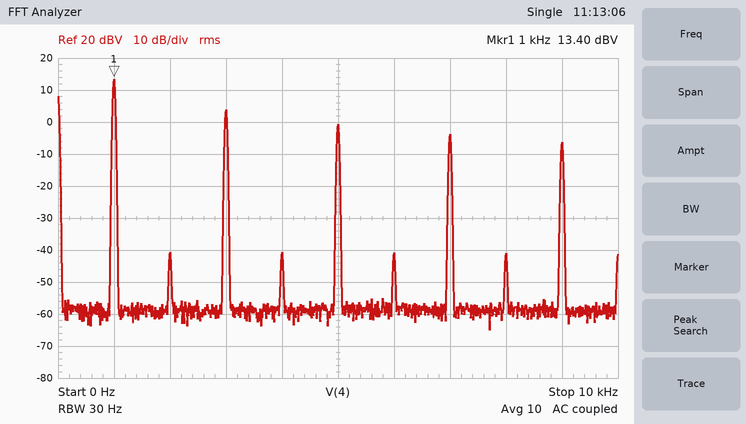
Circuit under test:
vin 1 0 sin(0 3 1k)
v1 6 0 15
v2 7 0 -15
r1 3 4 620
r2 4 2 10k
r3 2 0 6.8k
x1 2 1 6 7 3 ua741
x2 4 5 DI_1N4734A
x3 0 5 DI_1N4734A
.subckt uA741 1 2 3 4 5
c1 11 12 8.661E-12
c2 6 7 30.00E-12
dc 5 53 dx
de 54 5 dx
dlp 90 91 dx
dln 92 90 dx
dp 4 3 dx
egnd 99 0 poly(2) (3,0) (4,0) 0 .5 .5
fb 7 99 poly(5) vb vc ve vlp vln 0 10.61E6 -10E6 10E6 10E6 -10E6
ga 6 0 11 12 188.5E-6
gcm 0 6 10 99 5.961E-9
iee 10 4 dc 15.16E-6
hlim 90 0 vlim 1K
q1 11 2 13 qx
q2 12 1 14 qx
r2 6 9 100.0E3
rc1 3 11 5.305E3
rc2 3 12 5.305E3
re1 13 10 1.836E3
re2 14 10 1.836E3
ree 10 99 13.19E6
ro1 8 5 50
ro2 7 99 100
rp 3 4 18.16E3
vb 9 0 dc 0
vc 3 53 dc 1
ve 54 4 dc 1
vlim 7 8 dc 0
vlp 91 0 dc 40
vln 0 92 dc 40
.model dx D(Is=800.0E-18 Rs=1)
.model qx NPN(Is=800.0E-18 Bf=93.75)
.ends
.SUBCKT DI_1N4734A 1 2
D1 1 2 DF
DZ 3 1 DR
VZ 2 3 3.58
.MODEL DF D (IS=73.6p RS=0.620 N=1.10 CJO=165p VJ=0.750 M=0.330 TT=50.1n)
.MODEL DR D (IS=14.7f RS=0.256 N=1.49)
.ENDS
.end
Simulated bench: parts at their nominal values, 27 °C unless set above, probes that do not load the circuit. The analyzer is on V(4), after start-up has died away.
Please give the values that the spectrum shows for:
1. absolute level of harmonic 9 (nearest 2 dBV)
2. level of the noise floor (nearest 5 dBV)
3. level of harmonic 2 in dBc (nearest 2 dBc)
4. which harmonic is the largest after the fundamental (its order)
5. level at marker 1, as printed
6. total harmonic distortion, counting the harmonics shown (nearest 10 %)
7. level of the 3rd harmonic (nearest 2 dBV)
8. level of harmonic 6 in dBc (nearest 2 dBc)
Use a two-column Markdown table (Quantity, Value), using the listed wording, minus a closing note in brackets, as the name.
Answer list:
| Quantity | Value |
|---|---|
| absolute level of harmonic 9 | -6 dBV |
| level of the noise floor | -60 dBV |
| level of harmonic 2 in dBc | -54 dBc |
| which harmonic is the largest after the fundamental | 3 |
| level at marker 1, as printed | 13.40 dBV |
| total harmonic distortion, counting the harmonics shown | 40 % |
| level of the 3rd harmonic | 4 dBV |
| level of harmonic 6 in dBc | -54 dBc |
